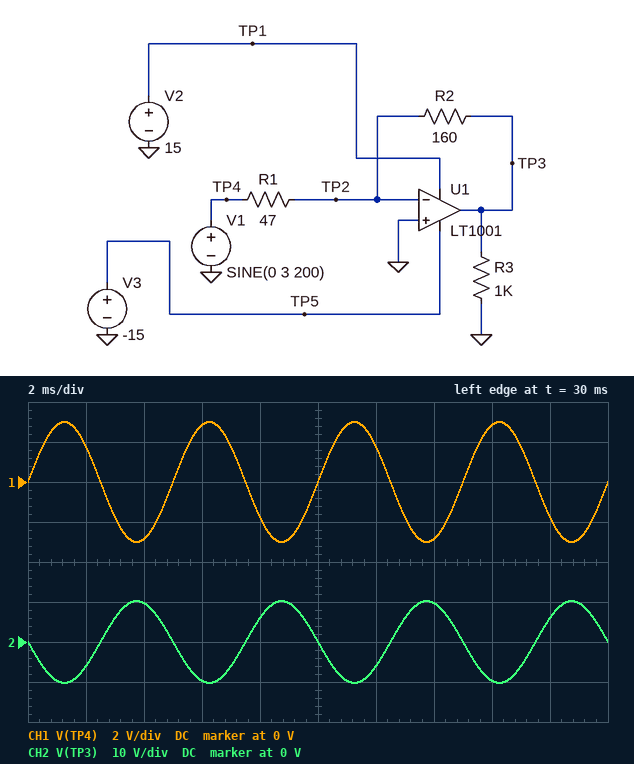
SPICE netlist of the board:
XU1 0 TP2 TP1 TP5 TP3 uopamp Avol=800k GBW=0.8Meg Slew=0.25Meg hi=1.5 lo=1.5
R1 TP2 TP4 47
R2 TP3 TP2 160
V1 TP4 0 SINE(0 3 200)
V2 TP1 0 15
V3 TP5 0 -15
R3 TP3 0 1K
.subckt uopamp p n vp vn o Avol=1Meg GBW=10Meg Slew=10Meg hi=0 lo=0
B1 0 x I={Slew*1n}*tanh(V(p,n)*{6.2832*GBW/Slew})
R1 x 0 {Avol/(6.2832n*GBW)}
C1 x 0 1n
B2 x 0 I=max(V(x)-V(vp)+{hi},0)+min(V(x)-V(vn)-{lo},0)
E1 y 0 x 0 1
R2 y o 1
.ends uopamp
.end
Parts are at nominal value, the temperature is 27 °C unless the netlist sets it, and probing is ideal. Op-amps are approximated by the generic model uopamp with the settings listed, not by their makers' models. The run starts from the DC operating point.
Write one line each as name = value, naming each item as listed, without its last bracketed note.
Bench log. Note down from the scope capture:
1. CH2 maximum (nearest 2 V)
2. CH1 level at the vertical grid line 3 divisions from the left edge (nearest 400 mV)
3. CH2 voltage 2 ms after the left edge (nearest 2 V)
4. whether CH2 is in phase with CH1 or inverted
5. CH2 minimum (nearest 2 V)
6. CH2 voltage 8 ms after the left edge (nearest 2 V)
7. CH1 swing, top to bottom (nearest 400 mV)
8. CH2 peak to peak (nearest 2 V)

CH2 maximum = 10 V
CH1 level at the vertical grid line 3 divisions from the left edge = 2.8 V
CH2 voltage 2 ms after the left edge = -6 V
whether CH2 is in phase with CH1 or inverted = inverted
CH2 minimum = -10 V
CH2 voltage 8 ms after the left edge = 6 V
CH1 swing, top to bottom = 6.0 V
CH2 peak to peak = 20 V
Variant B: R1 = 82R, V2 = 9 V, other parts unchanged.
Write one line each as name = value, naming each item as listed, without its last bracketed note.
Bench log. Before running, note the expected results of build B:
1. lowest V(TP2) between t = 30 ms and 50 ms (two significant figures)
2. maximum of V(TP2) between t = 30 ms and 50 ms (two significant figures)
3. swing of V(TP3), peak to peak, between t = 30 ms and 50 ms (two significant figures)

lowest V(TP2) between t = 30 ms and 50 ms = -1.5 mV
maximum of V(TP2) between t = 30 ms and 50 ms = 1.5 mV
swing of V(TP3), peak to peak, between t = 30 ms and 50 ms = 12 V
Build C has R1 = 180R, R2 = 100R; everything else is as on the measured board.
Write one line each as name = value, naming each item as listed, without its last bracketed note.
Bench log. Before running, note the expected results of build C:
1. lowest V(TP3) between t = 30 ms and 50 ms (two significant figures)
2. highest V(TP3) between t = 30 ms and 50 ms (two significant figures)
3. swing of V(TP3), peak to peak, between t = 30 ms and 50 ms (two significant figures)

lowest V(TP3) between t = 30 ms and 50 ms = -1.7 V
highest V(TP3) between t = 30 ms and 50 ms = 1.7 V
swing of V(TP3), peak to peak, between t = 30 ms and 50 ms = 3.3 V
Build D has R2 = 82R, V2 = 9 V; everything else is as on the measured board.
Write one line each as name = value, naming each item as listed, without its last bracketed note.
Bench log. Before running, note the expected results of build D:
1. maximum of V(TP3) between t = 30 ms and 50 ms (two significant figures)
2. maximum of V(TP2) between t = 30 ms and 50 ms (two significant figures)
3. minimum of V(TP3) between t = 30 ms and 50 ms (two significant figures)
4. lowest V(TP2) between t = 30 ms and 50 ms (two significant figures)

maximum of V(TP3) between t = 30 ms and 50 ms = 5.2 V
maximum of V(TP2) between t = 30 ms and 50 ms = 1.3 mV
minimum of V(TP3) between t = 30 ms and 50 ms = -5.2 V
lowest V(TP2) between t = 30 ms and 50 ms = -1.3 mV
